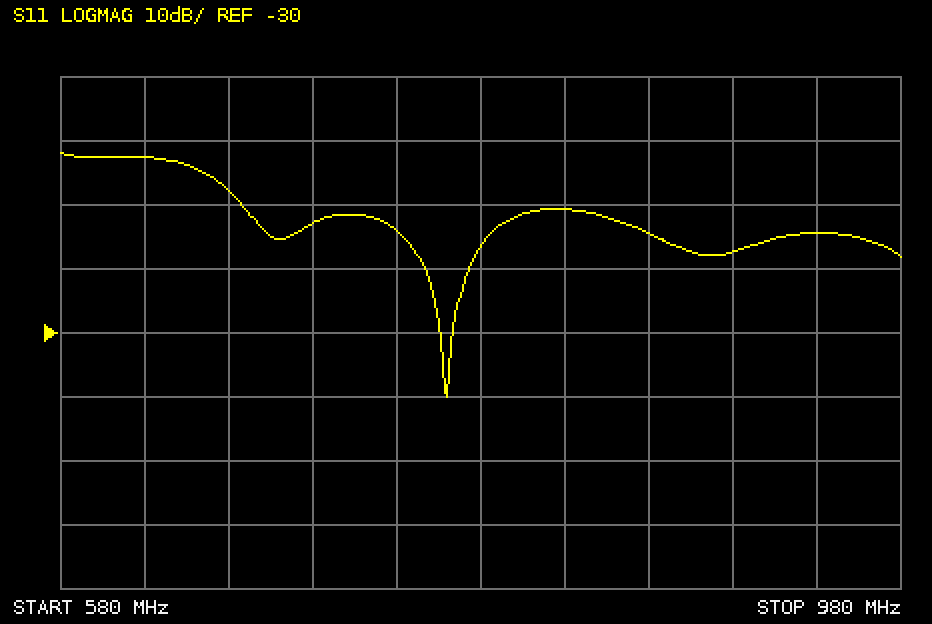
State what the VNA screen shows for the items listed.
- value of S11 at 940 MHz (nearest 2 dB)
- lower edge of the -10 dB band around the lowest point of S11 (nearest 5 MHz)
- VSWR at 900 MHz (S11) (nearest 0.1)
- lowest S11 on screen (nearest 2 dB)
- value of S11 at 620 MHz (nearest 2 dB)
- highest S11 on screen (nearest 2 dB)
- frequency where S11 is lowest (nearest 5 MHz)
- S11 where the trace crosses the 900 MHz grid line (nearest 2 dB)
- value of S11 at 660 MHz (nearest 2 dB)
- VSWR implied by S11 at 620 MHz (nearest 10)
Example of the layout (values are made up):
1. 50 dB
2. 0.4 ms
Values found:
1. -14 dB
2. 665 MHz
3. 1.3
4. -40 dB
5. -2 dB
6. -2 dB
7. 765 MHz
8. -18 dB
9. -8 dB
10. 10
